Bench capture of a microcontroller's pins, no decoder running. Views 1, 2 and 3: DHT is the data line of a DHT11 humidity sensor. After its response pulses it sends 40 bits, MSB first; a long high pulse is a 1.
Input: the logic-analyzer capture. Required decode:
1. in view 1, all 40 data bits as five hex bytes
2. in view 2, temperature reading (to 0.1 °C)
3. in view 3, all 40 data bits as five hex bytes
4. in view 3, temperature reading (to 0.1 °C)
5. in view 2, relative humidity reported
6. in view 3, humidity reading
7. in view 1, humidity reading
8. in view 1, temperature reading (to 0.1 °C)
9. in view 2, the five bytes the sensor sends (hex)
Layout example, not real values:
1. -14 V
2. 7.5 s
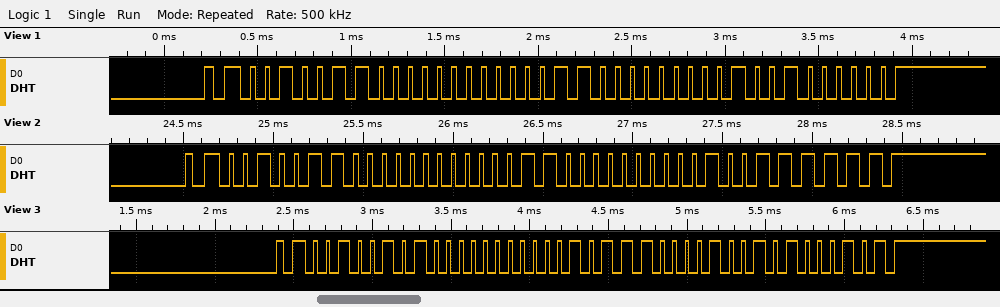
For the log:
1. 26 00 18 02 40
2. 24.1 °C
3. 25 00 17 09 45
4. 23.9 °C
5. 38 %
6. 37 %
7. 38 %
8. 24.2 °C
9. 26 00 18 01 3F
